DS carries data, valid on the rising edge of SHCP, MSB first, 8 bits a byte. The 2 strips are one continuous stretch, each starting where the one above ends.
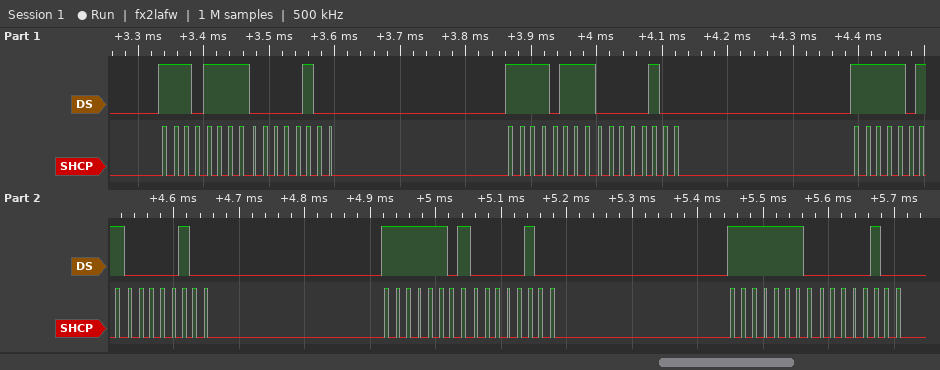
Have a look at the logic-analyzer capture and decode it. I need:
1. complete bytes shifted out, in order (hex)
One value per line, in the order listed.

EF 04 F7 04 FB 04 FD 04 FE 04
